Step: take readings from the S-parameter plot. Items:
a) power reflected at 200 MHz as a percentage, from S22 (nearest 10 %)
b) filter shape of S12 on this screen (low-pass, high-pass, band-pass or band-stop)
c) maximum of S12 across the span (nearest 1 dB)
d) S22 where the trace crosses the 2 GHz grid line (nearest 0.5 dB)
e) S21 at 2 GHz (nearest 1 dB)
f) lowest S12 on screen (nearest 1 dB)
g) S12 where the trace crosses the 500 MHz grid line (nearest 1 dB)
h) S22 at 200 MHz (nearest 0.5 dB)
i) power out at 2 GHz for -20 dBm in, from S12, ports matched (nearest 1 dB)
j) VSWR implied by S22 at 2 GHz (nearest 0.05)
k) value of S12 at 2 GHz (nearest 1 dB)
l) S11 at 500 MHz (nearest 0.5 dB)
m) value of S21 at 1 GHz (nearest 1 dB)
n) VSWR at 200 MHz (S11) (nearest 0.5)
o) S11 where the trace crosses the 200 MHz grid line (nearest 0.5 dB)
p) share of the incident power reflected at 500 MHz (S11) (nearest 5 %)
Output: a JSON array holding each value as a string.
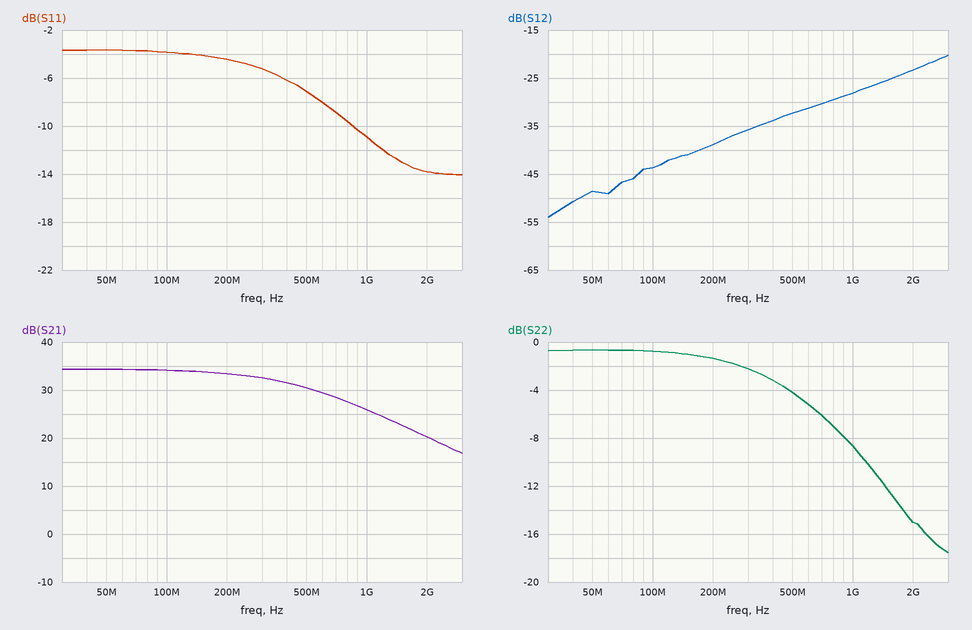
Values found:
["70 %", "high-pass", "-20 dB", "-15.0 dB", "20 dB", "-54 dB", "-32 dB", "-1.5 dB", "-43 dBm", "1.45", "-23 dB", "-7.0 dB", "26 dB", "4.0", "-4.5 dB", "20 %"]
